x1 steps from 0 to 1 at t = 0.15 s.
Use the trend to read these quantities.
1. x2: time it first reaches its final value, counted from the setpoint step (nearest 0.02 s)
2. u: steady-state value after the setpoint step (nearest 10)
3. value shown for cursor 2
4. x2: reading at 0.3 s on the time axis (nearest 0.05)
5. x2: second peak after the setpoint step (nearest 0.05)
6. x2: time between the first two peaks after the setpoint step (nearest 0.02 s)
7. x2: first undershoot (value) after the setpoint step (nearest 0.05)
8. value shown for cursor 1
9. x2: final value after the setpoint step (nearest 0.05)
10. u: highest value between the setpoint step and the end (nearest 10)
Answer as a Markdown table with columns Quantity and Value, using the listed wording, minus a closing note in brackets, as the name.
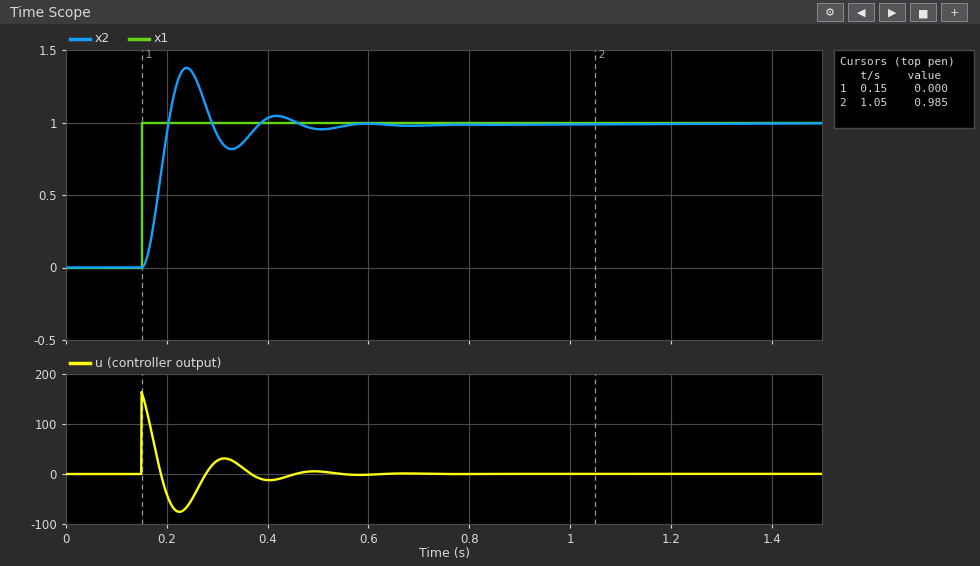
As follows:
| Quantity | Value |
|---|---|
| x2: time it first reaches its final value, counted from the setpoint step | 0.06 s |
| u: steady-state value after the setpoint step | 0 |
| value shown for cursor 2 | 0.985 |
| x2: reading at 0.3 s on the time axis | 0.90 |
| x2: second peak after the setpoint step | 1.05 |
| x2: time between the first two peaks after the setpoint step | 0.18 s |
| x2: first undershoot (value) after the setpoint step | 0.80 |
| value shown for cursor 1 | 0.000 |
| x2: final value after the setpoint step | 1.00 |
| u: highest value between the setpoint step and the end | 160 |
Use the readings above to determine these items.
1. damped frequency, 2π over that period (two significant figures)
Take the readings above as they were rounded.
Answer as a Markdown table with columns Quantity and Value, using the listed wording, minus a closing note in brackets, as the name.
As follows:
| Quantity | Value |
|---|---|
| damped frequency, 2π over that period | 35 rad/s |
